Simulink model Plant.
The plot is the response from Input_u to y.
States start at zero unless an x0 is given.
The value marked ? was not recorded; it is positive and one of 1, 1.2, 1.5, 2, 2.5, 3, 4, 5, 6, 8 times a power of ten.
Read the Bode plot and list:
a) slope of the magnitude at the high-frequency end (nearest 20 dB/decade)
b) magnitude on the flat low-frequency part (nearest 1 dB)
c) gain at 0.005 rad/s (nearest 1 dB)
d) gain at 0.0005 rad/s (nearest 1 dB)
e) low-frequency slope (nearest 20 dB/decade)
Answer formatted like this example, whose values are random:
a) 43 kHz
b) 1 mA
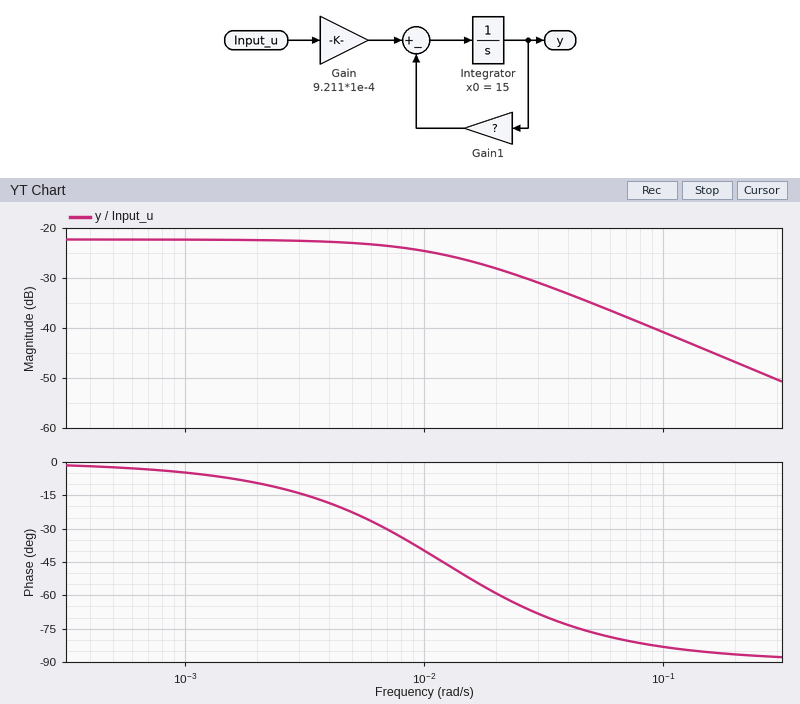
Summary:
a) -20 dB/decade
b) -22 dB
c) -23 dB
d) -22 dB
e) 0 dB/decade
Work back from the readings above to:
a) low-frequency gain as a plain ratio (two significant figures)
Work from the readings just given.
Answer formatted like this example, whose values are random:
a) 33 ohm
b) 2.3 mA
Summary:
a) 0.079
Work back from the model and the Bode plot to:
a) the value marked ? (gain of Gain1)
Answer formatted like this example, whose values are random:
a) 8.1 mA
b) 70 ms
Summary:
a) 0.012
